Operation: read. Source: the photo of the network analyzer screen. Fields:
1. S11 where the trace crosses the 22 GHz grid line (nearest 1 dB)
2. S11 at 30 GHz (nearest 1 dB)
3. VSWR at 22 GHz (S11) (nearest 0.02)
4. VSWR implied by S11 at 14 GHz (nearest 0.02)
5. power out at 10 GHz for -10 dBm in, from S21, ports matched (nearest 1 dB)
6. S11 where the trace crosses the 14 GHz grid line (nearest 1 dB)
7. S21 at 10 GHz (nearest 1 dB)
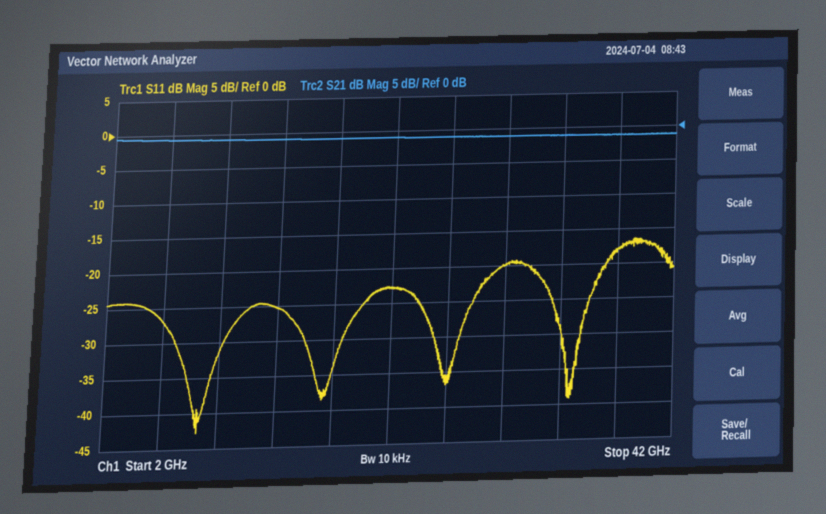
-23 dB
-20 dB
1.16
1.12
-11 dBm
-25 dB
-1 dB
